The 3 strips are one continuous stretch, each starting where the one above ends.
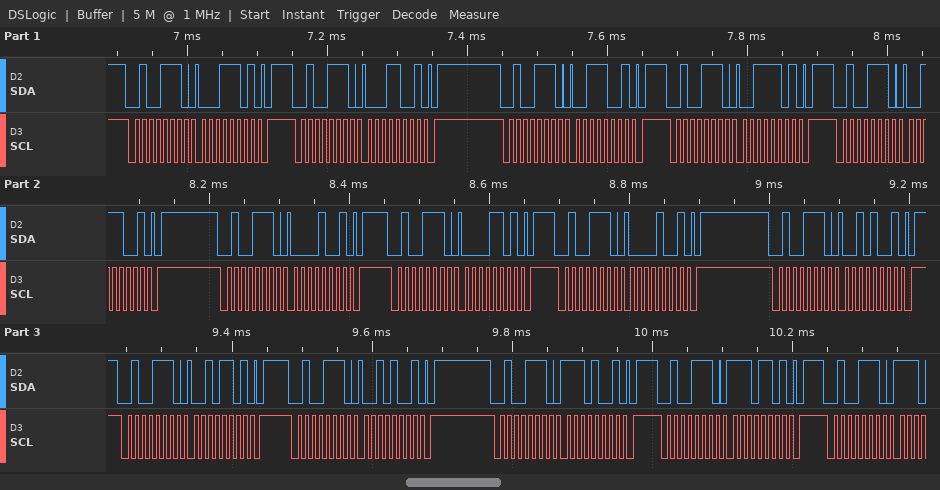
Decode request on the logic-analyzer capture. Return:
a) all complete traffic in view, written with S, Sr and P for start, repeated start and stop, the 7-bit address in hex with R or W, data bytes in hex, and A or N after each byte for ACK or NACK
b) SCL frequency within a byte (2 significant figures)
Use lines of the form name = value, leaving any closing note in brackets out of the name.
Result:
all complete traffic in view, written with S, Sr and P for start, repeated start and stop, the 7-bit address in hex with R or W, data bytes in hex, and A or N after each byte for ACK or NACK = S 27W A 1D A P S 27W A 19 A P S 27W A 39 A P S 27W A 3D A P S 27W A 39 A P S 27W A 09 A P S 27W A 0D A P S 27W A 09 A P S 27W A 29 A P S 27W A 2D A P S 27W A 29 A P S 27W A E9 A P S 27W A ED A P S 27W A
SCL frequency within a byte = 100 kHz
